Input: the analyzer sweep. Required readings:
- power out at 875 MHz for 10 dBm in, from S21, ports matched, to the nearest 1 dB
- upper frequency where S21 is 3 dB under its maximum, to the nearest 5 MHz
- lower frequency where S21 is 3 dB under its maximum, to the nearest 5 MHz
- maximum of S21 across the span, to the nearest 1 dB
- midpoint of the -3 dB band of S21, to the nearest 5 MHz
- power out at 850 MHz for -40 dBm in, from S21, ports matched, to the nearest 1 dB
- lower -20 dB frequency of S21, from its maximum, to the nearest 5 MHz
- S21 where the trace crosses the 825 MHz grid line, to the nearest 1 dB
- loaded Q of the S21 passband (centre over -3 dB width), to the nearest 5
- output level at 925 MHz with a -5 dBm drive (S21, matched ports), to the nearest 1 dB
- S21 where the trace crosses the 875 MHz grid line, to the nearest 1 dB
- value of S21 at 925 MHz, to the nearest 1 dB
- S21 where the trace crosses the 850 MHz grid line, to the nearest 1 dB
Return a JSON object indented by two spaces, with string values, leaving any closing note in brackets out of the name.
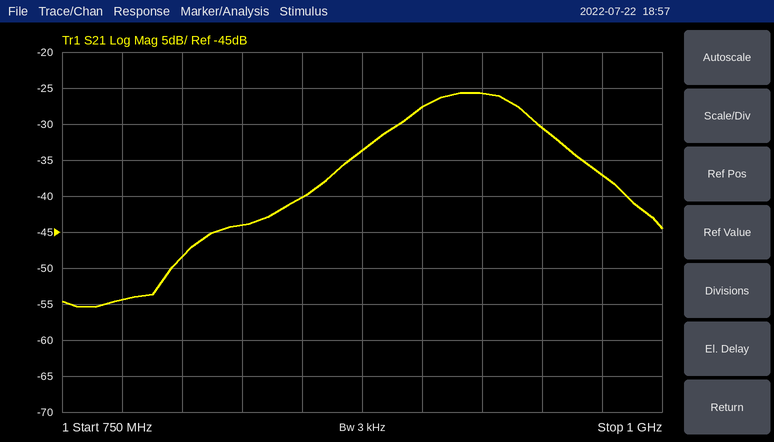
{
  "power out at 875 MHz for 10 dBm in, from S21, ports matched, to the nearest 1 dB": "-24 dBm",
  "upper frequency where S21 is 3 dB under its maximum, to the nearest 5 MHz": "945 MHz",
  "lower frequency where S21 is 3 dB under its maximum, to the nearest 5 MHz": "895 MHz",
  "maximum of S21 across the span, to the nearest 1 dB": "-26 dB",
  "midpoint of the -3 dB band of S21, to the nearest 5 MHz": "920 MHz",
  "power out at 850 MHz for -40 dBm in, from S21, ports matched, to the nearest 1 dB": "-80 dBm",
  "lower -20 dB frequency of S21, from its maximum, to the nearest 5 MHz": "810 MHz",
  "S21 where the trace crosses the 825 MHz grid line, to the nearest 1 dB": "-44 dB",
  "loaded Q of the S21 passband (centre over -3 dB width), to the nearest 5": "20",
  "output level at 925 MHz with a -5 dBm drive (S21, matched ports), to the nearest 1 dB": "-31 dBm",
  "S21 where the trace crosses the 875 MHz grid line, to the nearest 1 dB": "-34 dB",
  "value of S21 at 925 MHz, to the nearest 1 dB": "-26 dB",
  "S21 where the trace crosses the 850 MHz grid line, to the nearest 1 dB": "-40 dB"
}
